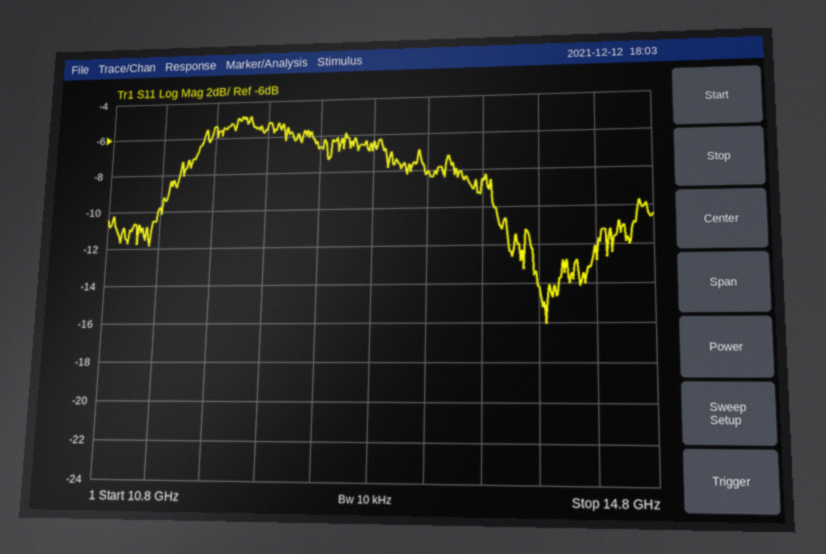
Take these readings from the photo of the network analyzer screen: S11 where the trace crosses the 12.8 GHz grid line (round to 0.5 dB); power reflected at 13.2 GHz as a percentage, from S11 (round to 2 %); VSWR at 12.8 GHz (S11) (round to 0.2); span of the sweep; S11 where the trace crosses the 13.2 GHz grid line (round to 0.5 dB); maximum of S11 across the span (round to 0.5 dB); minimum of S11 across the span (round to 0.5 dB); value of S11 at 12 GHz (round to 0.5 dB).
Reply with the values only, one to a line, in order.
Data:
-6.5 dB
16 %
2.8
4 GHz
-8.0 dB
-5.0 dB
-16.0 dB
-5.5 dB
